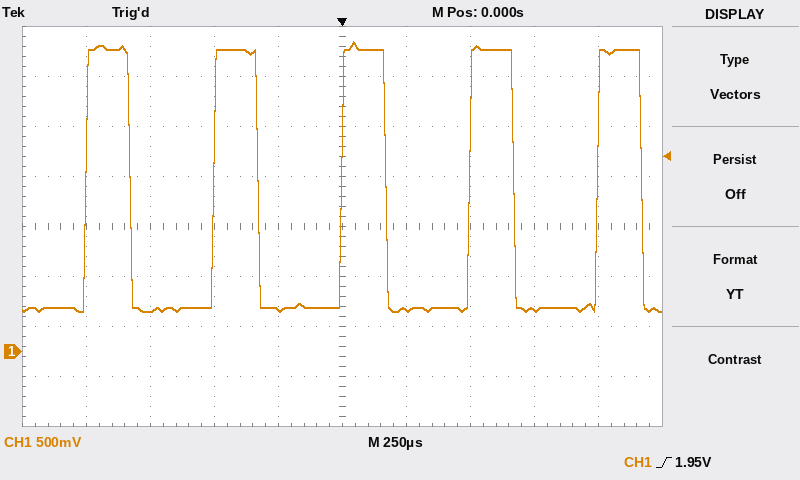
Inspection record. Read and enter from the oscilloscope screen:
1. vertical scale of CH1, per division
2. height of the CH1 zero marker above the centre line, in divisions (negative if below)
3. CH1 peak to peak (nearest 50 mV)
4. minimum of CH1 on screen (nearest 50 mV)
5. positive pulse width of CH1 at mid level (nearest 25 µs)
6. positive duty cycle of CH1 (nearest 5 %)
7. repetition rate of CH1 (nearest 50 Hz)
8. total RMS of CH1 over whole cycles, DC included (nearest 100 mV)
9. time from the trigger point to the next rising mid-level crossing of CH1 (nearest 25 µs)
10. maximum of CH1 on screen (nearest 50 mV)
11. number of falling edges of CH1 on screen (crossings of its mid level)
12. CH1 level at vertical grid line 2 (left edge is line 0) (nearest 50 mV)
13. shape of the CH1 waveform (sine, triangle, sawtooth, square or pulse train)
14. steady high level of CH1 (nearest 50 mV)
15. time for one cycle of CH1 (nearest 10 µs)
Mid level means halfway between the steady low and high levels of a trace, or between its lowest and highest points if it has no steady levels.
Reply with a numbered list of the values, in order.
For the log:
1. 500 mV
2. -2.5 div
3. 2.70 V
4. 400 mV
5. 175 µs
6. 35 %
7. 2.00 kHz
8. 1.8 V
9. 500 µs
10. 3.10 V
11. 5
12. 400 mV
13. pulse train
14. 3.00 V
15. 500 µs
